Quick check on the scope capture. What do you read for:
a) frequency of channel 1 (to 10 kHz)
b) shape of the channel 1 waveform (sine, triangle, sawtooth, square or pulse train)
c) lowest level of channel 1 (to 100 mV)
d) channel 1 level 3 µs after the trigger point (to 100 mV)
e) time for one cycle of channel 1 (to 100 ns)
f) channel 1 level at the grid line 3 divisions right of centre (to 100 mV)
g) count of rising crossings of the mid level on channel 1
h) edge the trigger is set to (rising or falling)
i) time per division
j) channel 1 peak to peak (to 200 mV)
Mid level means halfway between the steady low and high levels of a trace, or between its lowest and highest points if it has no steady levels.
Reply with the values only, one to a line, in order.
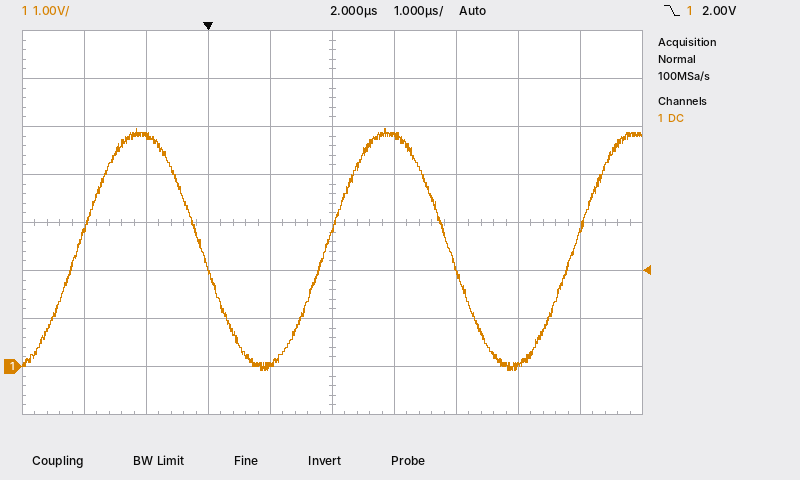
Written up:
250 kHz
sine
-100 mV
4.8 V
4.0 µs
0.0 V
3
falling
1 µs
5.0 V
